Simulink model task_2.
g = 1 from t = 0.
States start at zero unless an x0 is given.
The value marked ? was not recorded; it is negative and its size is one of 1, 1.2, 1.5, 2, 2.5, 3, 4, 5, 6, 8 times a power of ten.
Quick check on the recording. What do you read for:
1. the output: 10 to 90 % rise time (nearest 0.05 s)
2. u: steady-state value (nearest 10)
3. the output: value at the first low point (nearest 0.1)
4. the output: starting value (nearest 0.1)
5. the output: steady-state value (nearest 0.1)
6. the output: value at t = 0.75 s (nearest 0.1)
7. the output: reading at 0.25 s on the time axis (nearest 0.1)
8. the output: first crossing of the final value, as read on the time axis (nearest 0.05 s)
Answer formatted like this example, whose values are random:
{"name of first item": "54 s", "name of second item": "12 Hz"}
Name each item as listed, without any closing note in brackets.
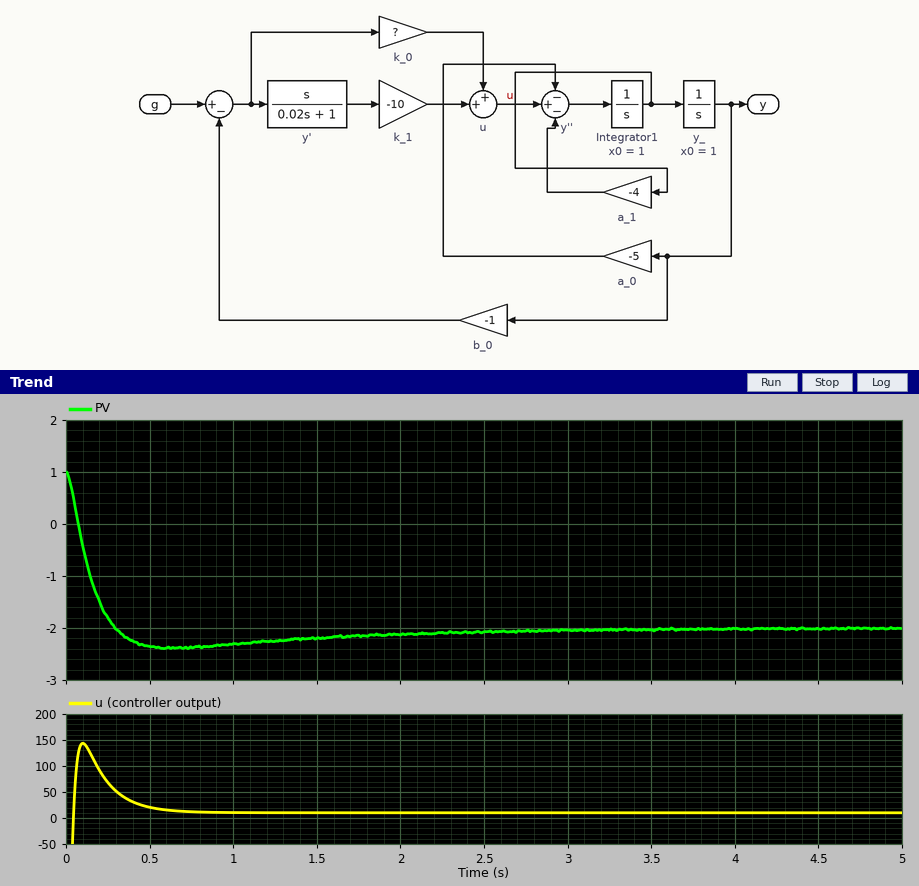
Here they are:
{"the output: 10 to 90 % rise time": "0.20 s", "u: steady-state value": "10", "the output: value at the first low point": "-2.4", "the output: starting value": "1.0", "the output: steady-state value": "-2.0", "the output: value at t = 0.75 s": "-2.4", "the output: reading at 0.25 s on the time axis": "-1.8", "the output: first crossing of the final value, as read on the time axis": "0.30 s"}
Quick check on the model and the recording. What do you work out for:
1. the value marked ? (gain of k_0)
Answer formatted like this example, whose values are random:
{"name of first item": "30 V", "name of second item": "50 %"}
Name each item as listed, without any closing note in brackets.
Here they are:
{"the value marked ?": "-10"}
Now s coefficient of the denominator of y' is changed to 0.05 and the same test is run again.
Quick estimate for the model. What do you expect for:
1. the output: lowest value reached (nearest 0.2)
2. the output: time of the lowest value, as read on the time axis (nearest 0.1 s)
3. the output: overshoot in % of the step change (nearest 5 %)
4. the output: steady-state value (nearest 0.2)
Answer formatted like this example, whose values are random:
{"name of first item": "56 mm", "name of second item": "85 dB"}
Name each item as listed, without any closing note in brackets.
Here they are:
{"the output: lowest value reached": "-2.6", "the output: time of the lowest value, as read on the time axis": "0.4 s", "the output: overshoot in % of the step change": "20 %", "the output: steady-state value": "-2.0"}
